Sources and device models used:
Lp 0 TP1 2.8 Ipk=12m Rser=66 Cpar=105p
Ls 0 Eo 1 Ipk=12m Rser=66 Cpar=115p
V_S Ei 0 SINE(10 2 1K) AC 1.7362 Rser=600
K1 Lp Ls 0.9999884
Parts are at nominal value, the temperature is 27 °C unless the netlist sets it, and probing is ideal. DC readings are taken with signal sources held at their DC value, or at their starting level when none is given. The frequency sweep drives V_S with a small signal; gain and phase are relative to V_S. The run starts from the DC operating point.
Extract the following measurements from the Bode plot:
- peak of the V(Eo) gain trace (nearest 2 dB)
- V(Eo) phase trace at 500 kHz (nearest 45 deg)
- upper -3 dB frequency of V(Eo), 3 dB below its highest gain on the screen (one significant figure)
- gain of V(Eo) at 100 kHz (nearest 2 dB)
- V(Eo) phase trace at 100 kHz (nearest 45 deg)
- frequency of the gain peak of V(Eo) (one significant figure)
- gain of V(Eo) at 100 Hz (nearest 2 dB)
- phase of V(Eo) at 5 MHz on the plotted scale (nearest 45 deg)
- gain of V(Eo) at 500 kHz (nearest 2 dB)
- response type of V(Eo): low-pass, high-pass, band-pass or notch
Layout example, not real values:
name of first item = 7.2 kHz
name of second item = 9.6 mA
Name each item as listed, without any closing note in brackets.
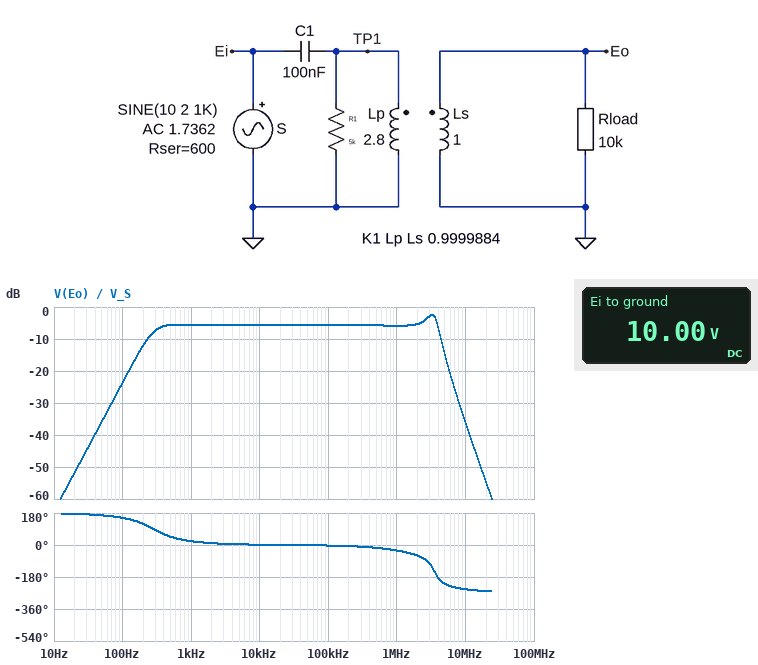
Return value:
peak of the V(Eo) gain trace = -2 dB
V(Eo) phase trace at 500 kHz = 0 deg
upper -3 dB frequency of V(Eo), 3 dB below its highest gain on the screen = 4 MHz
gain of V(Eo) at 100 kHz = -6 dB
V(Eo) phase trace at 100 kHz = 0 deg
frequency of the gain peak of V(Eo) = 3 MHz
gain of V(Eo) at 100 Hz = -24 dB
phase of V(Eo) at 5 MHz on the plotted scale = -225 deg
gain of V(Eo) at 500 kHz = -6 dB
response type of V(Eo): low-pass, high-pass, band-pass or notch = band-pass
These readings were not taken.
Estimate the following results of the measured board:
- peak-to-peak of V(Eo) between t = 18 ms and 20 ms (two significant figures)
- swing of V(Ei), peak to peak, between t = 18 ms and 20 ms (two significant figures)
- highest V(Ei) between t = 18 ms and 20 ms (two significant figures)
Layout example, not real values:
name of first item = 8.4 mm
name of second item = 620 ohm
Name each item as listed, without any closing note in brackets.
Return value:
peak-to-peak of V(Eo) between t = 18 ms and 20 ms = 2.1 V
swing of V(Ei), peak to peak, between t = 18 ms and 20 ms = 3.5 V
highest V(Ei) between t = 18 ms and 20 ms = 12 V
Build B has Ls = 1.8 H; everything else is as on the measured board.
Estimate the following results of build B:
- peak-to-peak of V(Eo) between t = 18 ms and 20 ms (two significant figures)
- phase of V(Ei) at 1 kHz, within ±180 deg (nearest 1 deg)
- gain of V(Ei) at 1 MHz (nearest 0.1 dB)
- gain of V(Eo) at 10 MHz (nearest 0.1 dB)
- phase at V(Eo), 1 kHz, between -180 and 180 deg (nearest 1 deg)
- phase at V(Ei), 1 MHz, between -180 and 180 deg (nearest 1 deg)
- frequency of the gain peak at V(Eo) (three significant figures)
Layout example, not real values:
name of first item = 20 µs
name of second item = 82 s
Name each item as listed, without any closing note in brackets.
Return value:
peak-to-peak of V(Eo) between t = 18 ms and 20 ms = 2.7 V
phase of V(Ei) at 1 kHz, within ±180 deg = -2 deg
gain of V(Ei) at 1 MHz = -3.0 dB
gain of V(Eo) at 10 MHz = -39.0 dB
phase at V(Eo), 1 kHz, between -180 and 180 deg = 23 deg
phase at V(Ei), 1 MHz, between -180 and 180 deg = -31 deg
frequency of the gain peak at V(Eo) = 2.48 MHz
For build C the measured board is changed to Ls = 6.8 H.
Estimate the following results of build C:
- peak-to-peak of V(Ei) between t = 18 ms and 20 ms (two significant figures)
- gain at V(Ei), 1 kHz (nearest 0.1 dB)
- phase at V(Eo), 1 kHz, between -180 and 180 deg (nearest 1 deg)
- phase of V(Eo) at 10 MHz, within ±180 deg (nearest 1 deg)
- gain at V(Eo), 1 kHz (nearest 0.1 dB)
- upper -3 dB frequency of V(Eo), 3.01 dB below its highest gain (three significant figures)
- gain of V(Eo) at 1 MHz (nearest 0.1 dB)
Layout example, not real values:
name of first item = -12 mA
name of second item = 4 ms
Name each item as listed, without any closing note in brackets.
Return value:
peak-to-peak of V(Ei) between t = 18 ms and 20 ms = 3.3 V
gain at V(Ei), 1 kHz = -1.6 dB
phase at V(Eo), 1 kHz, between -180 and 180 deg = 32 deg
phase of V(Eo) at 10 MHz, within ±180 deg = 109 deg
gain at V(Eo), 1 kHz = 0.8 dB
upper -3 dB frequency of V(Eo), 3.01 dB below its highest gain = 1.50 MHz
gain of V(Eo) at 1 MHz = 0.2 dB
